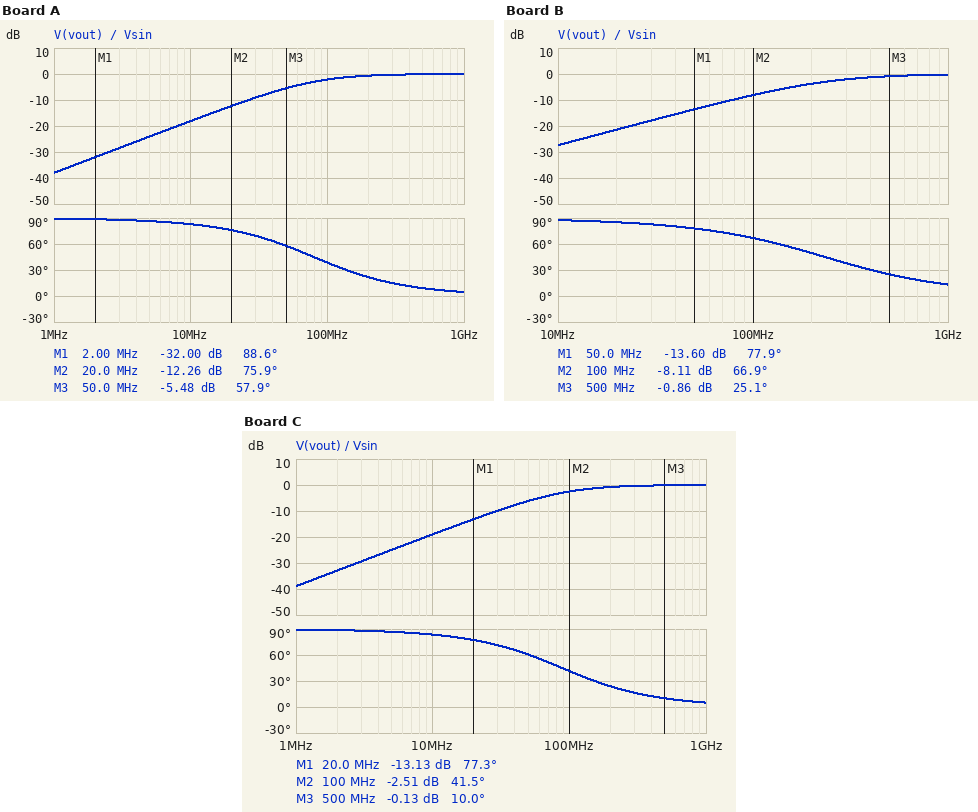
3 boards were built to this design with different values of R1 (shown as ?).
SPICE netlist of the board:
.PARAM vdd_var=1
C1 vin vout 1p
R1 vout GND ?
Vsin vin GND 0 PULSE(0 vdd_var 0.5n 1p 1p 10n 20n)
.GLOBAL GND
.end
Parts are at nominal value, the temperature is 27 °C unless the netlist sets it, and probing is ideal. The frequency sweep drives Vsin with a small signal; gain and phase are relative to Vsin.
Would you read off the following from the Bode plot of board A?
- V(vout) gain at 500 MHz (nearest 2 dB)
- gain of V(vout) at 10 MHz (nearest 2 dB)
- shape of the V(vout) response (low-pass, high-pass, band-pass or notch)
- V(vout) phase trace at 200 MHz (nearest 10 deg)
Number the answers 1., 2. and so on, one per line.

1. 0 dB
2. -18 dB
3. high-pass
4. 20 deg
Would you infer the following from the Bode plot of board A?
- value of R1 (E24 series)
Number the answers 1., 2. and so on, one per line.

1. 2 kΩ
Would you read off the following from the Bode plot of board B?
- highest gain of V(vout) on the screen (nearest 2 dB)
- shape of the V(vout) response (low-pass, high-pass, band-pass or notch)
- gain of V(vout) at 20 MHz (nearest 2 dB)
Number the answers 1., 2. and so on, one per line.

1. 0 dB
2. high-pass
3. -22 dB
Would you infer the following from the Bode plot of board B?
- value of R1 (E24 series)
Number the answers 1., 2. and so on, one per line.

1. 680 Ω
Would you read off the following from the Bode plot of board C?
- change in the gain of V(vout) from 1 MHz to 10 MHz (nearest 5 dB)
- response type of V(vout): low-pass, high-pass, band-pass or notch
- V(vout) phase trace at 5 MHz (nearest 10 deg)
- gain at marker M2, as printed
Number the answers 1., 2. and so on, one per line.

1. 20 dB
2. high-pass
3. 90 deg
4. -2.51 dB
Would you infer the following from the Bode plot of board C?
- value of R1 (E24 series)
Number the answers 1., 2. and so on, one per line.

1. 1.8 kΩ
